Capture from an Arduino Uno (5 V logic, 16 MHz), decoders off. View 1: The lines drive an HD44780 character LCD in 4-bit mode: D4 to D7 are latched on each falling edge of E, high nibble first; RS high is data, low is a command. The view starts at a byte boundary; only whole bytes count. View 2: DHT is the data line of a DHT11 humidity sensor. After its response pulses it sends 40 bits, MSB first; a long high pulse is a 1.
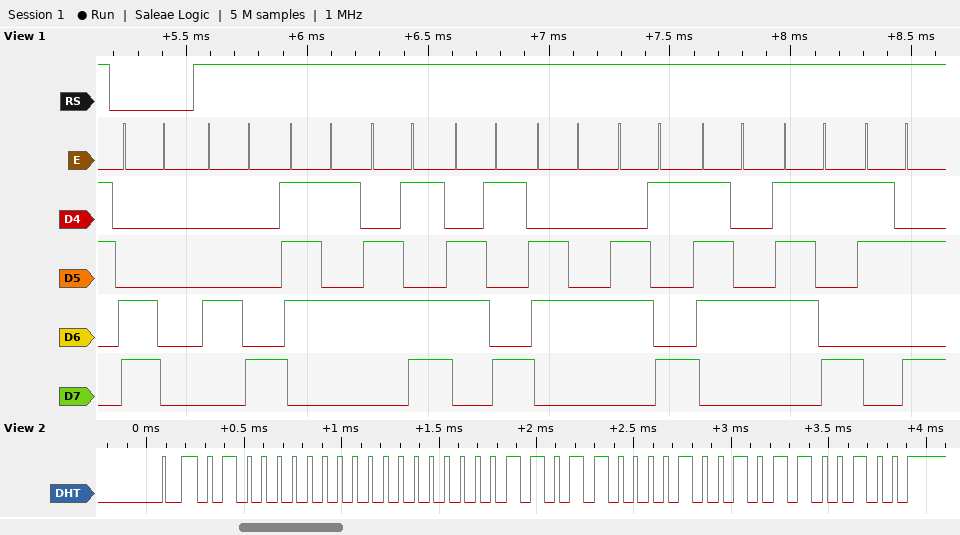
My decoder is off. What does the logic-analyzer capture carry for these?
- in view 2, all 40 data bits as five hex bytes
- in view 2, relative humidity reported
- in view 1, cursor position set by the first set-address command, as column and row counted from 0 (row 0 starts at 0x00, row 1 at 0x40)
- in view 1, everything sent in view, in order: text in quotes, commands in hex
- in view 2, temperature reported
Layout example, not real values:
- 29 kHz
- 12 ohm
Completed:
- 40 00 1B 09 64
- 64 %
- column 0, row 1
- 0xC0 "Humidity:"
- 27.9 °C
